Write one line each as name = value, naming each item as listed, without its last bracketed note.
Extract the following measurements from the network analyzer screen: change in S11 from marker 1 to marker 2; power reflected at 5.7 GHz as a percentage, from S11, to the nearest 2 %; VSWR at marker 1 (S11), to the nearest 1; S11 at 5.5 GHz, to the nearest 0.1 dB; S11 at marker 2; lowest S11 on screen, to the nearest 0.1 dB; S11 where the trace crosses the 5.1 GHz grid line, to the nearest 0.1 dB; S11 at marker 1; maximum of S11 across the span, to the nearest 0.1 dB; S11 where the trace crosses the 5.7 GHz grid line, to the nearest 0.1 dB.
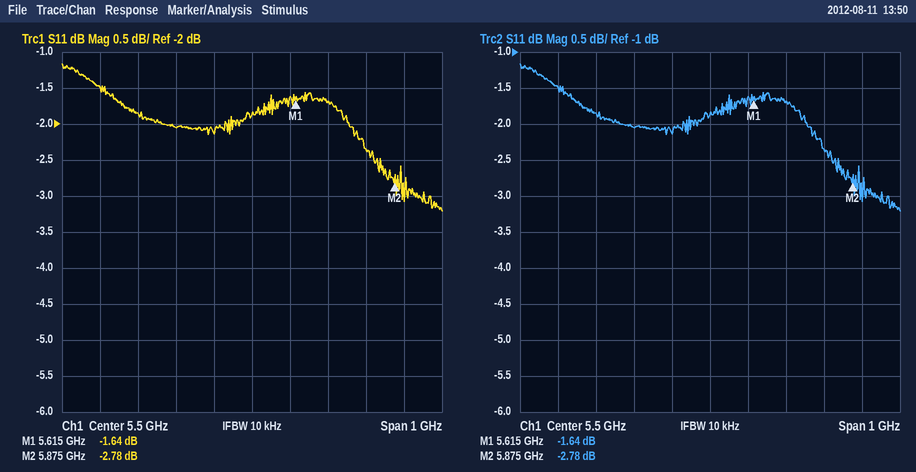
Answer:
change in S11 from marker 1 to marker 2 = -1.14 dB
power reflected at 5.7 GHz as a percentage, from S11, to the nearest 2 % = 68 %
VSWR at marker 1 (S11), to the nearest 1 = 11
S11 at 5.5 GHz, to the nearest 0.1 dB = -1.9 dB
S11 at marker 2 = -2.78 dB
lowest S11 on screen, to the nearest 0.1 dB = -3.2 dB
S11 where the trace crosses the 5.1 GHz grid line, to the nearest 0.1 dB = -1.5 dB
S11 at marker 1 = -1.64 dB
maximum of S11 across the span, to the nearest 0.1 dB = -1.2 dB
S11 where the trace crosses the 5.7 GHz grid line, to the nearest 0.1 dB = -1.7 dB
